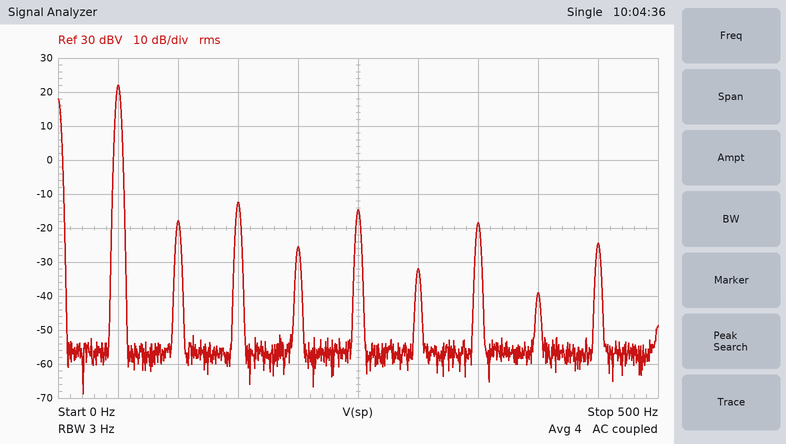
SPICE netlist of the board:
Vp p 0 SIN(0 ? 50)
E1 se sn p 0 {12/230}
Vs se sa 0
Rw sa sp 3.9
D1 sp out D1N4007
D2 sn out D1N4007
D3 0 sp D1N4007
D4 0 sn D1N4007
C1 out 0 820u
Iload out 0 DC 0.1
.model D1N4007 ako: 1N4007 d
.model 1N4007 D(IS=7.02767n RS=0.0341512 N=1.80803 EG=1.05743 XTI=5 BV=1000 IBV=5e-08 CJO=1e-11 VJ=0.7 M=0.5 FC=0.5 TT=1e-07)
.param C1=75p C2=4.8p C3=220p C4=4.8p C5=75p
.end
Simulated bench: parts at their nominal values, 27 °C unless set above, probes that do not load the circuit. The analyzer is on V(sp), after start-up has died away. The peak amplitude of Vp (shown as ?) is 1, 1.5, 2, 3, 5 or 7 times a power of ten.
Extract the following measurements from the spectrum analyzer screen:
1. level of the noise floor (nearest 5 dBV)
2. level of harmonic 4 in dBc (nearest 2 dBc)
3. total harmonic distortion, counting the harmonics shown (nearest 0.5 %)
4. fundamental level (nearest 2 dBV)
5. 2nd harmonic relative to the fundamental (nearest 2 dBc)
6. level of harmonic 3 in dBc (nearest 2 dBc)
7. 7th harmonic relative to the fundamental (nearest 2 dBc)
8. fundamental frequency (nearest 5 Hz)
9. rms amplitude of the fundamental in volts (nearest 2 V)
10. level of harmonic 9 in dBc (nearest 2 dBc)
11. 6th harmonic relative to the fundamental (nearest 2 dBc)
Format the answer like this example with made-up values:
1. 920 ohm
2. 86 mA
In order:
1. -55 dBV
2. -48 dBc
3. 3.0 %
4. 22 dBV
5. -40 dBc
6. -34 dBc
7. -40 dBc
8. 50 Hz
9. 12 V
10. -46 dBc
11. -54 dBc
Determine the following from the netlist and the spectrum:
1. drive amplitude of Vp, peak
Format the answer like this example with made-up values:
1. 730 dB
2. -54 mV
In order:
1. 700 V
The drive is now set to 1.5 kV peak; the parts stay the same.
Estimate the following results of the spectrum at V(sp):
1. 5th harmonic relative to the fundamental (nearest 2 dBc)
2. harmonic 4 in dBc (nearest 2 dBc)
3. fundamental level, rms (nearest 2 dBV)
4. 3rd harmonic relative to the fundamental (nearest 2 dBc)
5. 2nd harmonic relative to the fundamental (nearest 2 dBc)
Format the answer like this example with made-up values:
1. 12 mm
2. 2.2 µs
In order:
1. -42 dBc
2. -54 dBc
3. 28 dBV
4. -40 dBc
5. -46 dBc
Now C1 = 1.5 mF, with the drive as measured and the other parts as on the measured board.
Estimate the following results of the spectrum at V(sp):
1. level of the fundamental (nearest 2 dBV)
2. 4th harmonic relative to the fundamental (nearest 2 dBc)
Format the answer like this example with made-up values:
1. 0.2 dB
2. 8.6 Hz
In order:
1. 22 dBV
2. -52 dBc
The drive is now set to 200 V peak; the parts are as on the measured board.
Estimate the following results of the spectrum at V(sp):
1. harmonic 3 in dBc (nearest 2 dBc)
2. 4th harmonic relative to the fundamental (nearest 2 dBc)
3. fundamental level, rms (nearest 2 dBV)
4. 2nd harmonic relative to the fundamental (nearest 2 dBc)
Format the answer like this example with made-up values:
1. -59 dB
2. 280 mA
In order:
1. -24 dBc
2. -40 dBc
3. 10 dBV
4. -30 dBc
